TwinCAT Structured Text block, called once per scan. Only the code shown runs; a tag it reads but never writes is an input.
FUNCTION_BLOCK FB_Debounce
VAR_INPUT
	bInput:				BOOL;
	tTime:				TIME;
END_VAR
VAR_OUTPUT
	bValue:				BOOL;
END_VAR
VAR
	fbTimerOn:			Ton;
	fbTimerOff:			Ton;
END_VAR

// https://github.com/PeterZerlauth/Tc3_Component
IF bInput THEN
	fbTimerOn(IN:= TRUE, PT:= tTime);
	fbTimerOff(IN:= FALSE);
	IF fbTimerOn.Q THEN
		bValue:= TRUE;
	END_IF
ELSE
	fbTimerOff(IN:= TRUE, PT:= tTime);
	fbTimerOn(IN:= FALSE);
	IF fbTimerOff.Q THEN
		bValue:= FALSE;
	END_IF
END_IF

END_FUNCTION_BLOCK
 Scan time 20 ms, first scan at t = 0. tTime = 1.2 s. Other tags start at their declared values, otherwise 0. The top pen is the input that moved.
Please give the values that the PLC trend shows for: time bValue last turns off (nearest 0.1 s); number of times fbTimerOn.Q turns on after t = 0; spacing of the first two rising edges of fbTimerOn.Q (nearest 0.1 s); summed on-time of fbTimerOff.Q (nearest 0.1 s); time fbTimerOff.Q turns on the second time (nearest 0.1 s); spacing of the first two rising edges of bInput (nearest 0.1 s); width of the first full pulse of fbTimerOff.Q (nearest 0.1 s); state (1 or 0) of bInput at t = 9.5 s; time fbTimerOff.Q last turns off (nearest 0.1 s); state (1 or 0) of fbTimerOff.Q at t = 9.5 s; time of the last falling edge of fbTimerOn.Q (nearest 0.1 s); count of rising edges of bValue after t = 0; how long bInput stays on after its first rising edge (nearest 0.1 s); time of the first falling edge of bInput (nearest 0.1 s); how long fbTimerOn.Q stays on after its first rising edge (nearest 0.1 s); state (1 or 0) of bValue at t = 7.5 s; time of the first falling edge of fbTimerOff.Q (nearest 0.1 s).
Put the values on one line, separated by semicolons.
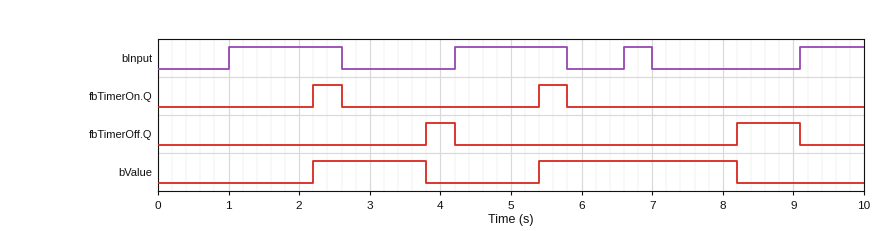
8.2 s; 2; 3.2 s; 1.3 s; 8.2 s; 3.2 s; 0.4 s; 1; 9.1 s; 0; 5.8 s; 2; 1.6 s; 2.6 s; 0.4 s; 1; 4.2 s
